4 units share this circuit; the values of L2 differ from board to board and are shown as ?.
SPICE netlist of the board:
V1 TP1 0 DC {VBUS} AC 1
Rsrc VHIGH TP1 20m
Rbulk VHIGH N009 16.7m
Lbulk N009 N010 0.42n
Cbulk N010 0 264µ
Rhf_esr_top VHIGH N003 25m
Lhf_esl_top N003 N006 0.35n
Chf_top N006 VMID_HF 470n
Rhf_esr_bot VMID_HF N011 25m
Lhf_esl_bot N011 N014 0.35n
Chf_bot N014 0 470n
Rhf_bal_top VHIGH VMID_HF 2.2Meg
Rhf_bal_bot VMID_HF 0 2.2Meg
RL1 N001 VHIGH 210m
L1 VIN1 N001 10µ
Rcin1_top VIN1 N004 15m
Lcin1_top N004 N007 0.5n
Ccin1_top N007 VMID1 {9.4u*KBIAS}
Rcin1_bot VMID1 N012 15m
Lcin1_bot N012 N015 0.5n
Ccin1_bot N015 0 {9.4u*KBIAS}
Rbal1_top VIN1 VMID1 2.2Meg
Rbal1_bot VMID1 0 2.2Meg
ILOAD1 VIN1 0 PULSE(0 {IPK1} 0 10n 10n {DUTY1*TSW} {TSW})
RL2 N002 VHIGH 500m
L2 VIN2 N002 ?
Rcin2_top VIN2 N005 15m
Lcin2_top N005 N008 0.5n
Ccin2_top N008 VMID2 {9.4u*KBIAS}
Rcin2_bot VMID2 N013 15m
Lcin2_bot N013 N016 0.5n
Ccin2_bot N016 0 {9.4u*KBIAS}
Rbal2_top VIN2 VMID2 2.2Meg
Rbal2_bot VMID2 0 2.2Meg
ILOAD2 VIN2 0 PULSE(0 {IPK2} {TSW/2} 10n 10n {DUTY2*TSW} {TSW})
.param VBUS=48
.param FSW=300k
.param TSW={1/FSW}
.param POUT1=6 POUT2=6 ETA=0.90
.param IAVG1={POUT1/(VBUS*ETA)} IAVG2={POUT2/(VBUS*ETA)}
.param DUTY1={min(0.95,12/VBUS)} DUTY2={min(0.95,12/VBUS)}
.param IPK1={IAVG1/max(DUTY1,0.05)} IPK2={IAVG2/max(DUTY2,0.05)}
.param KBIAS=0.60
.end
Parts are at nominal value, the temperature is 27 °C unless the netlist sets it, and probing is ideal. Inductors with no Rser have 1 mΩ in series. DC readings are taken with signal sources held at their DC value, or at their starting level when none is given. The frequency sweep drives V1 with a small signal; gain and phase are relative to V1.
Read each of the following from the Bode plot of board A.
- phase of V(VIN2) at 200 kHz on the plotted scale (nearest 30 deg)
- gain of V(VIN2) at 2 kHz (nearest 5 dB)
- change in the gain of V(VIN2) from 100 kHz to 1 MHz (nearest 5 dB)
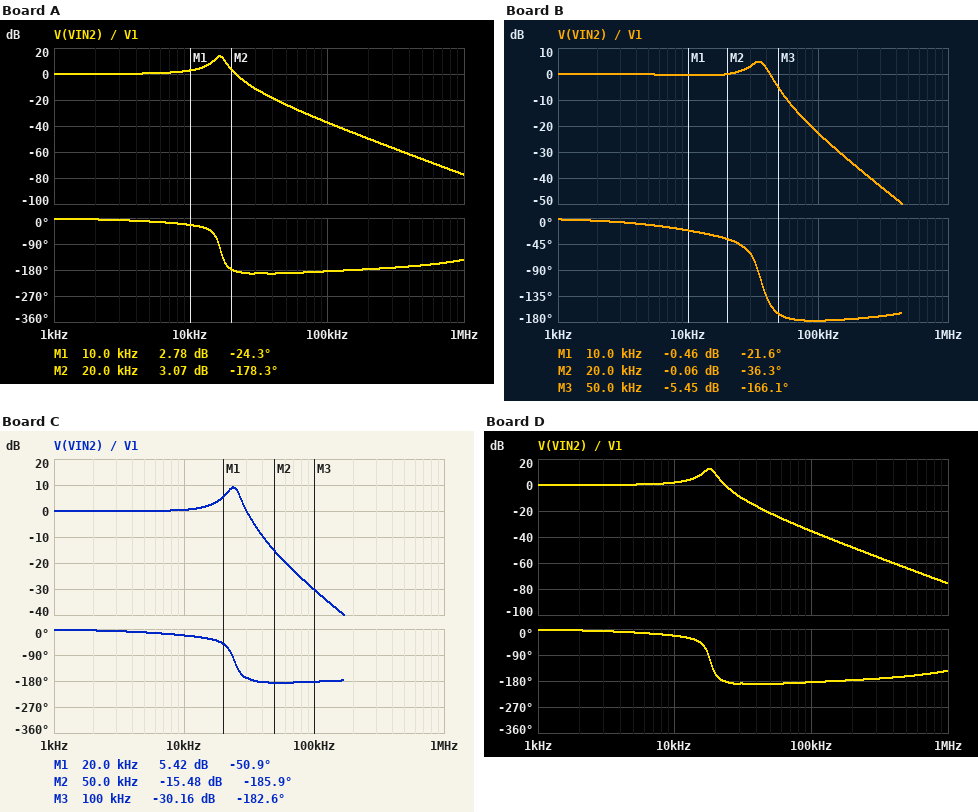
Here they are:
-180 deg
0 dB
-40 dB
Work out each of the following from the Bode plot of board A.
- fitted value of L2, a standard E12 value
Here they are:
33 µH
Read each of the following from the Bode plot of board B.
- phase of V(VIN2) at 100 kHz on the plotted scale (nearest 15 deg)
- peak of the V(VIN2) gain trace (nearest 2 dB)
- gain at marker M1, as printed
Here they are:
-180 deg
4 dB
-0.46 dB
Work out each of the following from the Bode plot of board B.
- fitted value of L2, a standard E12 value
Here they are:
6.8 µH
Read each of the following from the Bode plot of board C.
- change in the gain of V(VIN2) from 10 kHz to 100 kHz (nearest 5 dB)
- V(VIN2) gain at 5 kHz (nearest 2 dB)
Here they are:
-30 dB
0 dB
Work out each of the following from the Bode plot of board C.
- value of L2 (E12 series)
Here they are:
15 µH
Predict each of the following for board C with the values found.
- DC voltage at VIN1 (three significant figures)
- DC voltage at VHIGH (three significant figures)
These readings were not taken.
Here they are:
48.0 V
48.0 V
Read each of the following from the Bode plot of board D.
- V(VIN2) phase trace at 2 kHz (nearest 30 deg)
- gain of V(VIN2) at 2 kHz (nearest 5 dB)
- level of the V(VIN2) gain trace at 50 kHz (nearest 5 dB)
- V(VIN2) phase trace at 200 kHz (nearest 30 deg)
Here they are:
0 deg
0 dB
-20 dB
-180 deg
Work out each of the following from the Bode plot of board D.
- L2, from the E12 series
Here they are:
27 µH
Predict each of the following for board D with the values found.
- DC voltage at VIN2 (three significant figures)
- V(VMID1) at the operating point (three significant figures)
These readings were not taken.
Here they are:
48.0 V
24.0 V
